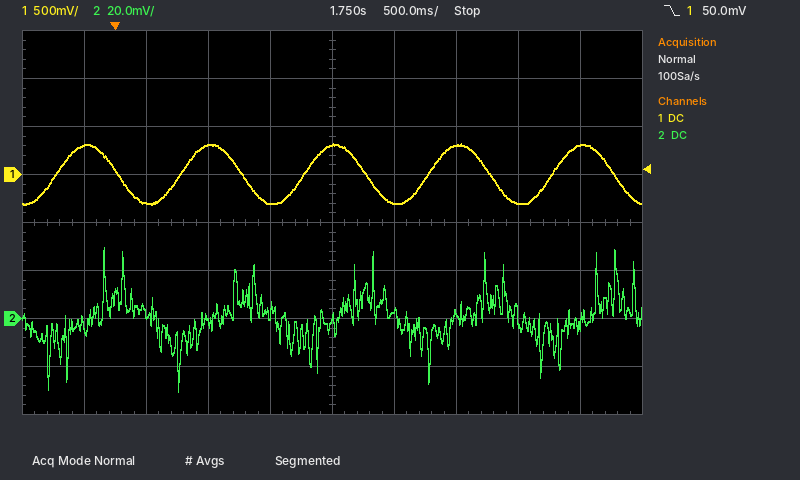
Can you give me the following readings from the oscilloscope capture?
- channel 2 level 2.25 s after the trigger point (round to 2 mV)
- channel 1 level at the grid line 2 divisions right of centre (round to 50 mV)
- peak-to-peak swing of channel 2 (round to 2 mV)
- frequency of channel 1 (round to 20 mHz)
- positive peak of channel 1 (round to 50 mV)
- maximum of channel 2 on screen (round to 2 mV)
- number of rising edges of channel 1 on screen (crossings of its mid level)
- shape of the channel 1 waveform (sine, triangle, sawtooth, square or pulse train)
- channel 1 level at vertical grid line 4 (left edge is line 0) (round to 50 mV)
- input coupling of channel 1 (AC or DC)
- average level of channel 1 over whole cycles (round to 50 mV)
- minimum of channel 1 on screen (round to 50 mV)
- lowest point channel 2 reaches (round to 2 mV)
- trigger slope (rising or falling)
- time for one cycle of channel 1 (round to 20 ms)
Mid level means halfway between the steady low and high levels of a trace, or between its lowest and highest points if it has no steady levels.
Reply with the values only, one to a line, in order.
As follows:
2 mV
300 mV
60 mV
1.00 Hz
300 mV
30 mV
5
sine
-300 mV
DC
0 mV
-300 mV
-30 mV
falling
1.00 s
